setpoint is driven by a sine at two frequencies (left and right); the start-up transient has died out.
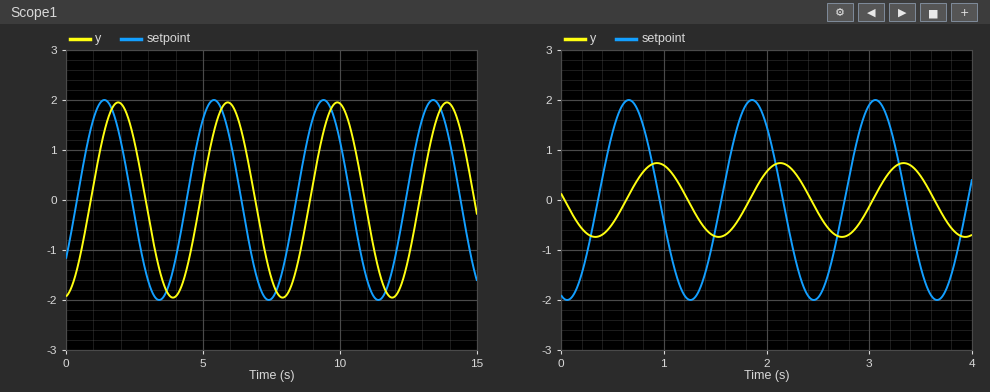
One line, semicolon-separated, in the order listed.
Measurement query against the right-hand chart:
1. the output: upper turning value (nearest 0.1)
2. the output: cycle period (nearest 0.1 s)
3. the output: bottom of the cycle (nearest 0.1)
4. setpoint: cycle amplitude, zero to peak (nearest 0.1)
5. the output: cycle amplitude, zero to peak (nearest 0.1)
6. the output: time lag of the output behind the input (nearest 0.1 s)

0.7; 1.2 s; -0.7; 2.0; 0.7; 0.3 s
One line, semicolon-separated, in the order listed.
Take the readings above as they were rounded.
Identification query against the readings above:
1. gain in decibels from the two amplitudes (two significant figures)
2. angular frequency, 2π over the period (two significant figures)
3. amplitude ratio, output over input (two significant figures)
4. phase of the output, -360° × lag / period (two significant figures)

-9.1 dB; 5.2 rad/s; 0.35; -90°
